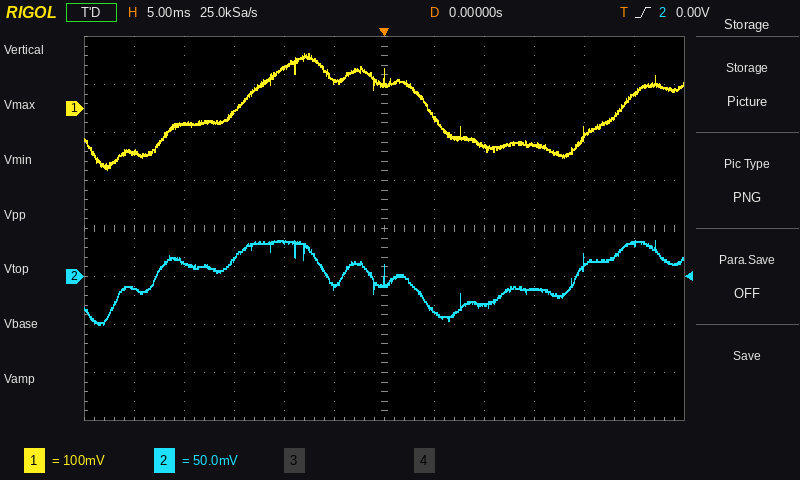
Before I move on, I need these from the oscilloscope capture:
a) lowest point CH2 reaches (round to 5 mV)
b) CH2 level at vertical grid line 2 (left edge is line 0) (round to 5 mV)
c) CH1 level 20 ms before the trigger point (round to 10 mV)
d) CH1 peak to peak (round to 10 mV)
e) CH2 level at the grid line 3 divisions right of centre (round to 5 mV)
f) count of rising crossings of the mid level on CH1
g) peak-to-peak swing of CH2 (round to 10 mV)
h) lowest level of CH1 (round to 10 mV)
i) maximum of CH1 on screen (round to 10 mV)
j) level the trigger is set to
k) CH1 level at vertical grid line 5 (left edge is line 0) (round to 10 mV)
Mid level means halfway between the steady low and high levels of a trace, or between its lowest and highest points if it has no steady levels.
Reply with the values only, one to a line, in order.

-50 mV
15 mV
-30 mV
240 mV
-15 mV
2
90 mV
-130 mV
110 mV
0.00 V
60 mV
